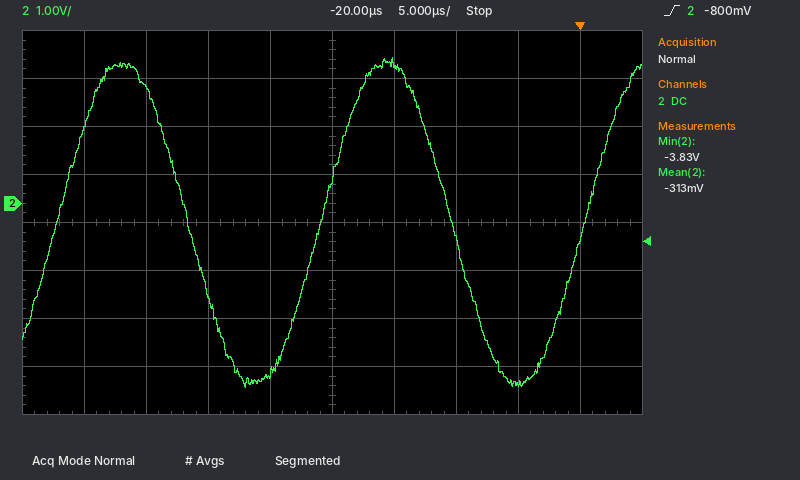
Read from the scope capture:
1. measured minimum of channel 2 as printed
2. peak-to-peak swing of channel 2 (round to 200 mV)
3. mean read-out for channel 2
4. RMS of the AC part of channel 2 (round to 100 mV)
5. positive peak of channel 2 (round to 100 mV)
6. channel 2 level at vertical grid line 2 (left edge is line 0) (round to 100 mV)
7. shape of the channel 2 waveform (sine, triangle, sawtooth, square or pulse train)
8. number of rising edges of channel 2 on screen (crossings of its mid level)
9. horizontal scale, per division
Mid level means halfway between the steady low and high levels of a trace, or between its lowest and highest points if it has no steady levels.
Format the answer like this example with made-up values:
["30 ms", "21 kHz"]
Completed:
["-3.83 V", "6.8 V", "-313 mV", "2.4 V", "3.0 V", "2.4 V", "sine", "3", "5 µs"]
